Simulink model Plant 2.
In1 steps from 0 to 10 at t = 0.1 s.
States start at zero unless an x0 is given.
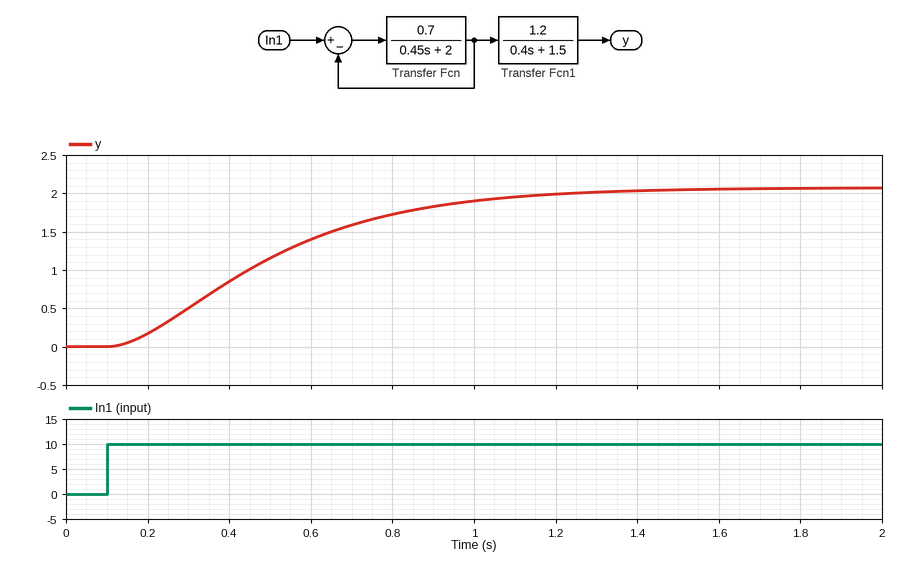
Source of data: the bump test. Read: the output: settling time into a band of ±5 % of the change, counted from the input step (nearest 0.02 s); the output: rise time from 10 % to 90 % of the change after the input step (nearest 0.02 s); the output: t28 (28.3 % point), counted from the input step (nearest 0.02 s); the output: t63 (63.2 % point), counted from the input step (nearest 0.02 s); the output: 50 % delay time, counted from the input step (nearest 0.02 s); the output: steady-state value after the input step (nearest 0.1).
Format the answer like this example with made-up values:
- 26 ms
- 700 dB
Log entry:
- 1.04 s
- 0.74 s
- 0.22 s
- 0.46 s
- 0.36 s
- 2.1
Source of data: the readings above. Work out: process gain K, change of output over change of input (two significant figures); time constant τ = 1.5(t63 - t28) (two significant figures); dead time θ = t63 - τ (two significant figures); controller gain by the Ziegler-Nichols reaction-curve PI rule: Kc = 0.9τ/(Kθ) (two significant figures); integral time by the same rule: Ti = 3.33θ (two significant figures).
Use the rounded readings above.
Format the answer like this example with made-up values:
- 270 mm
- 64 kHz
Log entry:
- 0.21
- 0.36 s
- 0.10 s
- 15
- 0.33 s
